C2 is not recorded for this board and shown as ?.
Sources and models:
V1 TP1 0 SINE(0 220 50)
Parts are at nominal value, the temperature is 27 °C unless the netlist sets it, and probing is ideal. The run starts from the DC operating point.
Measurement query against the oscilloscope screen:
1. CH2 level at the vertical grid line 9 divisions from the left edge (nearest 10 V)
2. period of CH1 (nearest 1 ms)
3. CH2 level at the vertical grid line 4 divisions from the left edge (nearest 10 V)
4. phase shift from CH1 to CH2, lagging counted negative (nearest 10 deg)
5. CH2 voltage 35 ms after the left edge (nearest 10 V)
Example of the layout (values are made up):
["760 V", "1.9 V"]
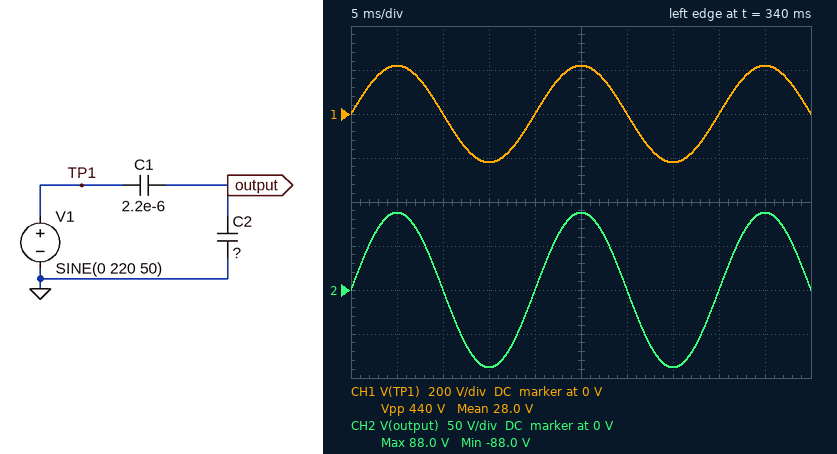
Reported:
["90 V", "20 ms", "0 V", "0 deg", "-90 V"]
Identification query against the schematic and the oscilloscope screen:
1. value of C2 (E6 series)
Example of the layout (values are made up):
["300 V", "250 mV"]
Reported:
["3.3 µF"]
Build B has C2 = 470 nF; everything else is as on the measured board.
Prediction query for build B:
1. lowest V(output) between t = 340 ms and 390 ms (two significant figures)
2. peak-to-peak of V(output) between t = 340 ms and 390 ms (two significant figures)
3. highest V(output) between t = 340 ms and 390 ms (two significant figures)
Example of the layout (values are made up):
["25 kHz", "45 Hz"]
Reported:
["-180 V", "360 V", "180 V"]
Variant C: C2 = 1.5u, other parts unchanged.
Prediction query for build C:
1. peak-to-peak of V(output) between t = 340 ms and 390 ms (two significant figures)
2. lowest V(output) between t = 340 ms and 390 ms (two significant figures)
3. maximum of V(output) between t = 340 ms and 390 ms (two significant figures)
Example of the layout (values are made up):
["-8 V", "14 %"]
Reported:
["260 V", "-130 V", "130 V"]
